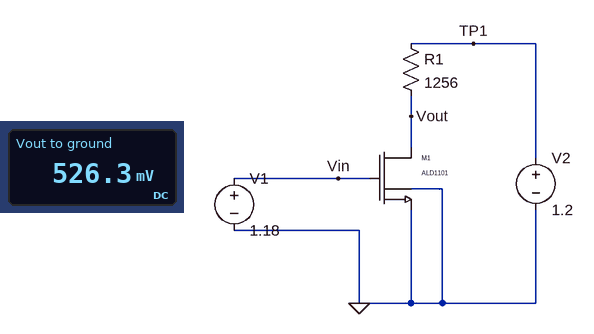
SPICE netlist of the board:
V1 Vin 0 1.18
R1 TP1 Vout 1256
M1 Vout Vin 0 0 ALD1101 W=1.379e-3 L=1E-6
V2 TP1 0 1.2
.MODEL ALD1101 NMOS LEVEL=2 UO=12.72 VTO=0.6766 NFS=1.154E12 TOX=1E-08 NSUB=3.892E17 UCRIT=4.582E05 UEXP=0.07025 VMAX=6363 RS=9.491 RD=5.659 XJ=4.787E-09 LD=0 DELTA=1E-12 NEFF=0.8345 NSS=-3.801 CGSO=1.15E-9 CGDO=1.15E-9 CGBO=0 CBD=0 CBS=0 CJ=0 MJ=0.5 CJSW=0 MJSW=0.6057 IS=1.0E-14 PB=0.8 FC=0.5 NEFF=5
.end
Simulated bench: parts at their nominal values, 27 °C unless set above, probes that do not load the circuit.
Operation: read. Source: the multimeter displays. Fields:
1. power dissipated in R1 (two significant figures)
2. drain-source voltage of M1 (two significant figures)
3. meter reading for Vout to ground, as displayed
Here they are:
360 µW
530 mV
526.3 mV
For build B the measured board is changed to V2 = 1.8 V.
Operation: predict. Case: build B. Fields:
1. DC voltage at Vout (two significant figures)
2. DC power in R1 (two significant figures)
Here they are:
1.1 V
370 µW
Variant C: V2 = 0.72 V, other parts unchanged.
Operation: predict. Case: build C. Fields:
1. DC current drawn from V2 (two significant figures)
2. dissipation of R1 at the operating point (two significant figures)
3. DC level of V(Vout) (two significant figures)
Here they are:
420 µA
220 µW
190 mV
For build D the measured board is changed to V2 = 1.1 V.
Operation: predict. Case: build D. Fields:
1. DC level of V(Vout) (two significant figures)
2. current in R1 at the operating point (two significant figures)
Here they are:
430 mV
530 µA
